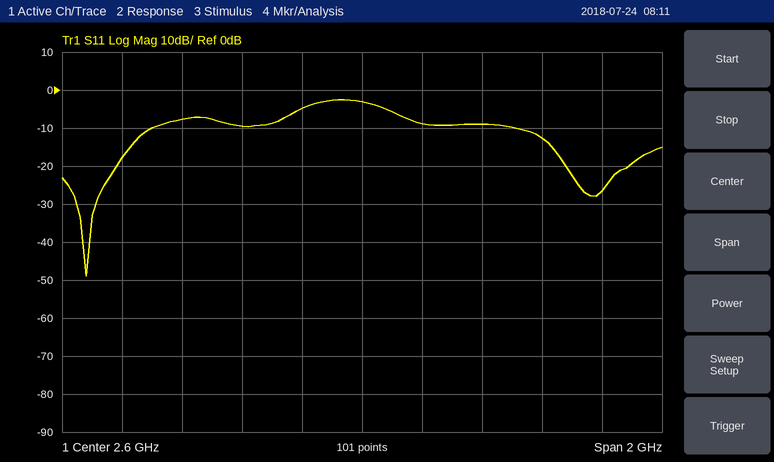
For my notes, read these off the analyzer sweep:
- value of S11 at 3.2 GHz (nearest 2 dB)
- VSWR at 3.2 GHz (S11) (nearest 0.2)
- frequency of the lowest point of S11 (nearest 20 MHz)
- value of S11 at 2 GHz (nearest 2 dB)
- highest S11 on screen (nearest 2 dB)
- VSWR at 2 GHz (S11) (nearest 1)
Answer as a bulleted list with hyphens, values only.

- -12 dB
- 1.6
- 1.68 GHz
- -8 dB
- -2 dB
- 2
